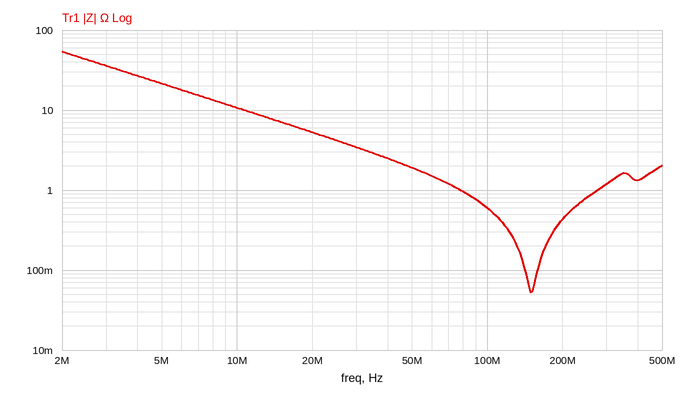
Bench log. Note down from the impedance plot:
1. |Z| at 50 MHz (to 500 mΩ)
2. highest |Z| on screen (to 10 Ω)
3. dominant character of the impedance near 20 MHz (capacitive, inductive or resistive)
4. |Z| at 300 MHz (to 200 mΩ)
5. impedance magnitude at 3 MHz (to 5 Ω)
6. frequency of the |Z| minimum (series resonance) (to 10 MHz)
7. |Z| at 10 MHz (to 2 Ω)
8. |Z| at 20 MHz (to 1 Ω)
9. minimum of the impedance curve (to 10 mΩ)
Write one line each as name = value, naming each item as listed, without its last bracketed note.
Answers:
|Z| at 50 MHz = 2.0 Ω
highest |Z| on screen = 50 Ω
dominant character of the impedance near 20 MHz = capacitive
|Z| at 300 MHz = 1.2 Ω
impedance magnitude at 3 MHz = 35 Ω
frequency of the |Z| minimum (series resonance) = 150 MHz
|Z| at 10 MHz = 10 Ω
|Z| at 20 MHz = 5 Ω
minimum of the impedance curve = 50 mΩ
